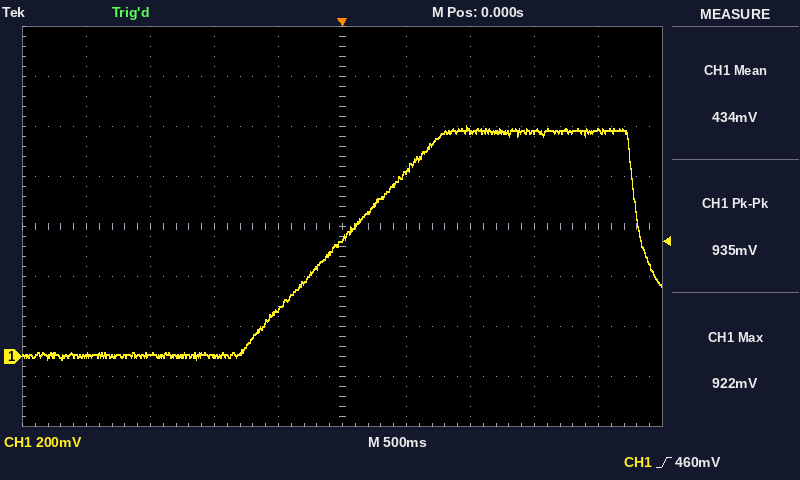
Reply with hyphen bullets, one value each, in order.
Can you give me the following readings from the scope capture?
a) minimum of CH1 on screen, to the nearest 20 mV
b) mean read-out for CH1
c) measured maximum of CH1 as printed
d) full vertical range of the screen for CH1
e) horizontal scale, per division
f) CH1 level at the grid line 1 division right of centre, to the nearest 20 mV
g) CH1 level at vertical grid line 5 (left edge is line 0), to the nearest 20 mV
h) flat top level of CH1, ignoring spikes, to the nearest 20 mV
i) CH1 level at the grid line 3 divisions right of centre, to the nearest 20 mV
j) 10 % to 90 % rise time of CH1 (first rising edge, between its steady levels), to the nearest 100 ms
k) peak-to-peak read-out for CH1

- -20 mV
- 434 mV
- 922 mV
- 1.6 V
- 500 ms
- 740 mV
- 480 mV
- 900 mV
- 900 mV
- 1.3 s
- 935 mV
